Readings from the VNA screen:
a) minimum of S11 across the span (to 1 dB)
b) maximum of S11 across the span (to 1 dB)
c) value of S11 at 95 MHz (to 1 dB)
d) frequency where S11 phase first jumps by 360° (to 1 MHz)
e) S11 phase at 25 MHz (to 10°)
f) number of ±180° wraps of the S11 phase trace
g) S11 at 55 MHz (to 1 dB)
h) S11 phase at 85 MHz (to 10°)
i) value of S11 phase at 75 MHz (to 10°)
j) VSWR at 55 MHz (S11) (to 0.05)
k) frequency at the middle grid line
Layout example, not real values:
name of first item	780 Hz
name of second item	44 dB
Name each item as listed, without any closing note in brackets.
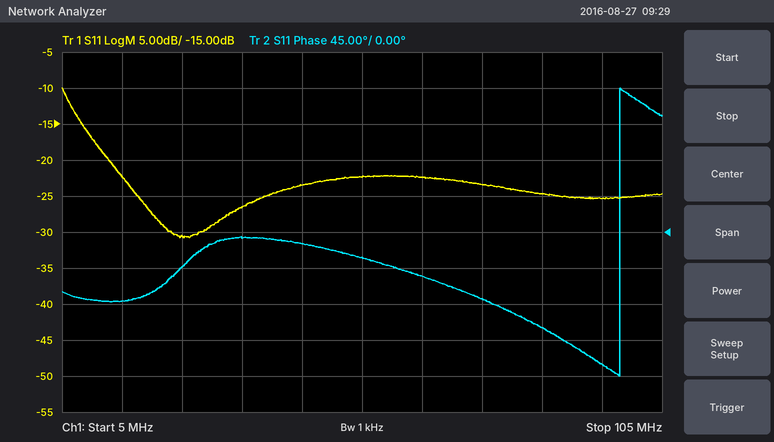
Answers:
minimum of S11 across the span	-31 dB
maximum of S11 across the span	-10 dB
value of S11 at 95 MHz	-25 dB
frequency where S11 phase first jumps by 360°	98 MHz
S11 phase at 25 MHz	-40°
number of ±180° wraps of the S11 phase trace	1
S11 at 55 MHz	-22 dB
S11 phase at 85 MHz	-120°
value of S11 phase at 75 MHz	-80°
VSWR at 55 MHz (S11)	1.15
frequency at the middle grid line	55 MHz
